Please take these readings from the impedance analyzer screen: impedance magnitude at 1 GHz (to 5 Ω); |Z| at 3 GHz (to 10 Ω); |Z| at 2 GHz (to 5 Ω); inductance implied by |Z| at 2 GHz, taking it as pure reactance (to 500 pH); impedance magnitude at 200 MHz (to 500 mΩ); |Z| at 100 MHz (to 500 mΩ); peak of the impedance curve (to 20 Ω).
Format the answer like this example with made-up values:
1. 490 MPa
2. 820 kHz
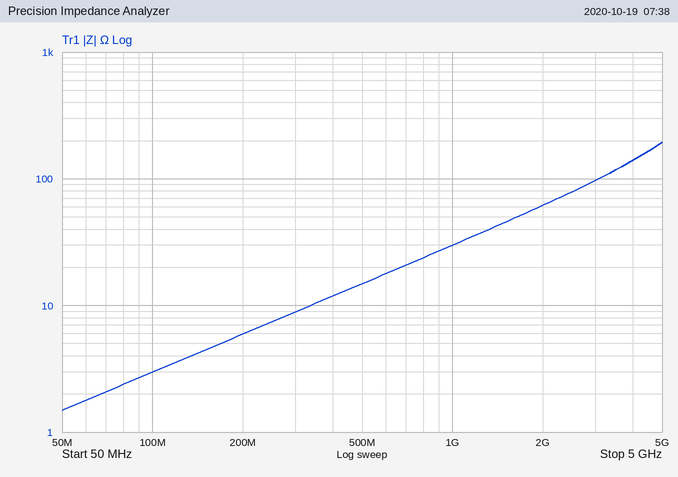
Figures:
1. 30 Ω
2. 100 Ω
3. 60 Ω
4. 5.0 nH
5. 6.0 Ω
6. 3.0 Ω
7. 200 Ω
